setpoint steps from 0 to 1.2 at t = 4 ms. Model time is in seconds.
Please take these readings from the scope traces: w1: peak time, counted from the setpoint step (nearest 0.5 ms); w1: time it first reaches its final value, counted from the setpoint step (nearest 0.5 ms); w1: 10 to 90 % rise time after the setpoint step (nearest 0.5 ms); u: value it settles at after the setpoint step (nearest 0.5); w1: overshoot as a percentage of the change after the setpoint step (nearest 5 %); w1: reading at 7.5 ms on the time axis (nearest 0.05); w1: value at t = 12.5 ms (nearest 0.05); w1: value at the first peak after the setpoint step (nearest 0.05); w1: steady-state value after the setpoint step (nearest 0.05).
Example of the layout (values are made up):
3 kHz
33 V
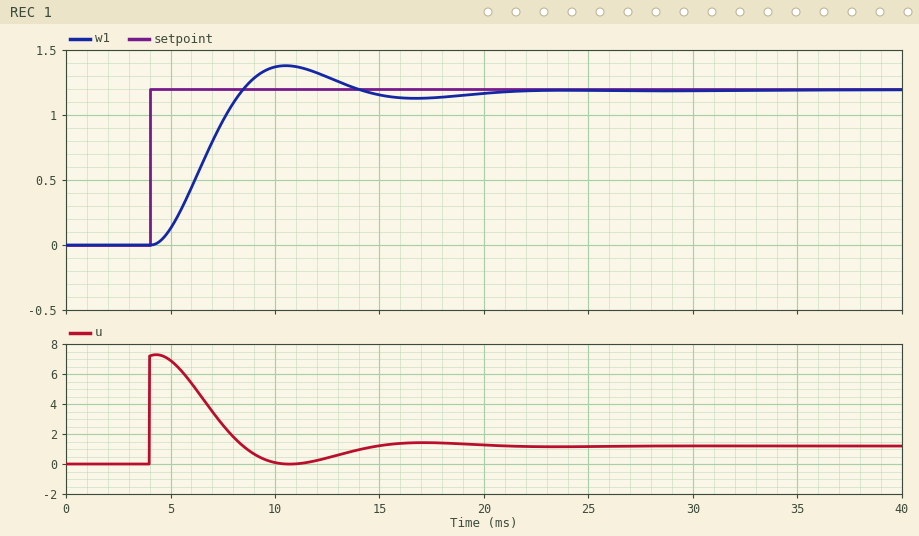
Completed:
6.5 ms
4.5 ms
3.0 ms
1.0
15 %
0.95
1.30
1.40
1.20
